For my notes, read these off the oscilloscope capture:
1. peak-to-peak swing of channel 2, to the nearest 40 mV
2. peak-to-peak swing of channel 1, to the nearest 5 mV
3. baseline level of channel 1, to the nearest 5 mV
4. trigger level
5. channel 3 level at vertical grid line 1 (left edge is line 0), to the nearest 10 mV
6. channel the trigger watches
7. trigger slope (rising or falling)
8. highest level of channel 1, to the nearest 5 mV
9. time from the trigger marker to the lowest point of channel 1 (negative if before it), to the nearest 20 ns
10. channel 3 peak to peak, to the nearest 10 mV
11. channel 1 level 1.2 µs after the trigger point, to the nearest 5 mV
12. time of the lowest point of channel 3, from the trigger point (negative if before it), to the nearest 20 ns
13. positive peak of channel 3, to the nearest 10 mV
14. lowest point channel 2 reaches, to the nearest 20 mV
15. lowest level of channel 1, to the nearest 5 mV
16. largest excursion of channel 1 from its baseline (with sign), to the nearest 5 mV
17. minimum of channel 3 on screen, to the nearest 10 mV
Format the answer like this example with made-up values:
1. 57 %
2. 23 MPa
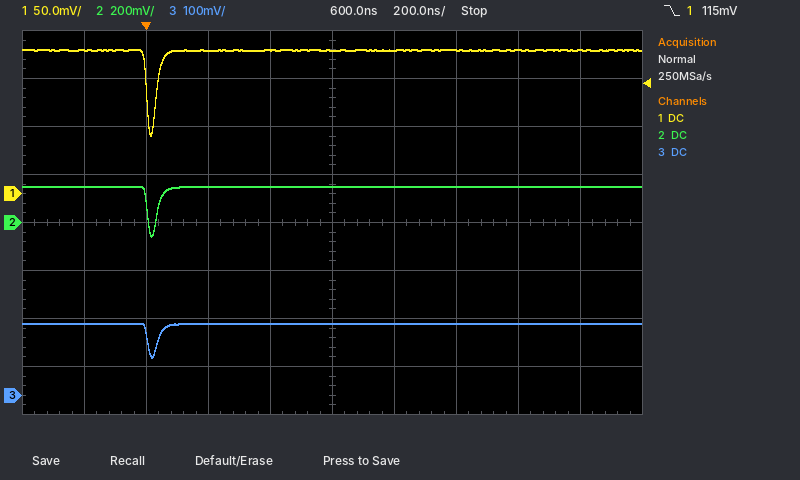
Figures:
1. 200 mV
2. 90 mV
3. 150 mV
4. 115 mV
5. 150 mV
6. channel 1
7. falling
8. 150 mV
9. +20 ns
10. 70 mV
11. 150 mV
12. +20 ns
13. 150 mV
14. -60 mV
15. 60 mV
16. -90 mV
17. 80 mV
